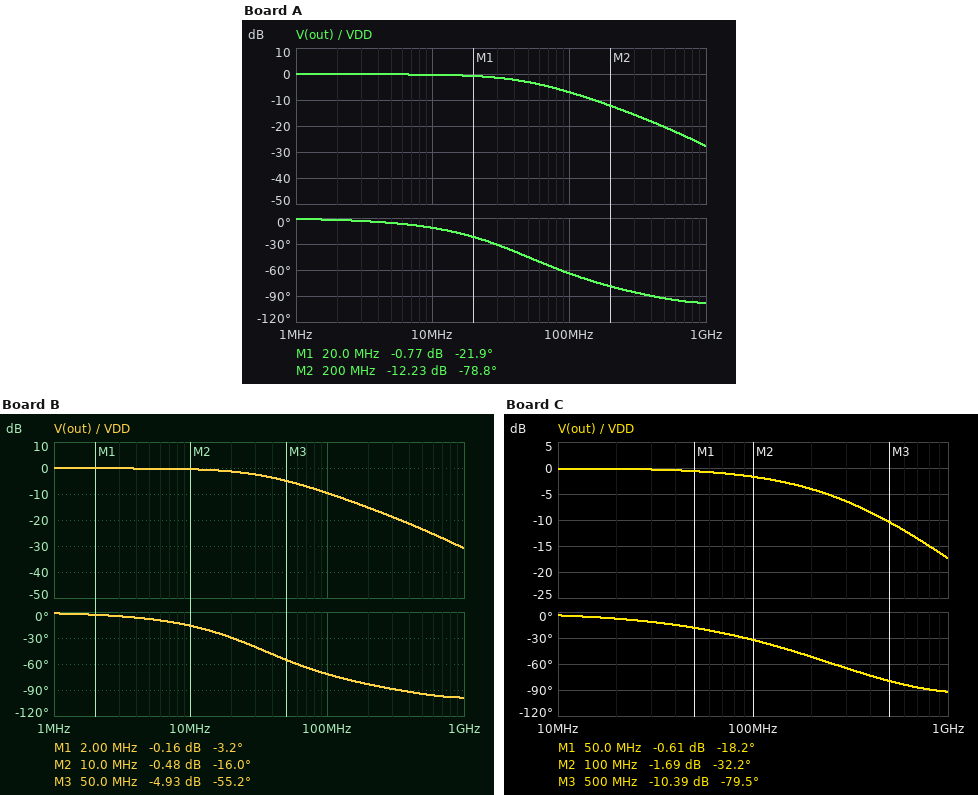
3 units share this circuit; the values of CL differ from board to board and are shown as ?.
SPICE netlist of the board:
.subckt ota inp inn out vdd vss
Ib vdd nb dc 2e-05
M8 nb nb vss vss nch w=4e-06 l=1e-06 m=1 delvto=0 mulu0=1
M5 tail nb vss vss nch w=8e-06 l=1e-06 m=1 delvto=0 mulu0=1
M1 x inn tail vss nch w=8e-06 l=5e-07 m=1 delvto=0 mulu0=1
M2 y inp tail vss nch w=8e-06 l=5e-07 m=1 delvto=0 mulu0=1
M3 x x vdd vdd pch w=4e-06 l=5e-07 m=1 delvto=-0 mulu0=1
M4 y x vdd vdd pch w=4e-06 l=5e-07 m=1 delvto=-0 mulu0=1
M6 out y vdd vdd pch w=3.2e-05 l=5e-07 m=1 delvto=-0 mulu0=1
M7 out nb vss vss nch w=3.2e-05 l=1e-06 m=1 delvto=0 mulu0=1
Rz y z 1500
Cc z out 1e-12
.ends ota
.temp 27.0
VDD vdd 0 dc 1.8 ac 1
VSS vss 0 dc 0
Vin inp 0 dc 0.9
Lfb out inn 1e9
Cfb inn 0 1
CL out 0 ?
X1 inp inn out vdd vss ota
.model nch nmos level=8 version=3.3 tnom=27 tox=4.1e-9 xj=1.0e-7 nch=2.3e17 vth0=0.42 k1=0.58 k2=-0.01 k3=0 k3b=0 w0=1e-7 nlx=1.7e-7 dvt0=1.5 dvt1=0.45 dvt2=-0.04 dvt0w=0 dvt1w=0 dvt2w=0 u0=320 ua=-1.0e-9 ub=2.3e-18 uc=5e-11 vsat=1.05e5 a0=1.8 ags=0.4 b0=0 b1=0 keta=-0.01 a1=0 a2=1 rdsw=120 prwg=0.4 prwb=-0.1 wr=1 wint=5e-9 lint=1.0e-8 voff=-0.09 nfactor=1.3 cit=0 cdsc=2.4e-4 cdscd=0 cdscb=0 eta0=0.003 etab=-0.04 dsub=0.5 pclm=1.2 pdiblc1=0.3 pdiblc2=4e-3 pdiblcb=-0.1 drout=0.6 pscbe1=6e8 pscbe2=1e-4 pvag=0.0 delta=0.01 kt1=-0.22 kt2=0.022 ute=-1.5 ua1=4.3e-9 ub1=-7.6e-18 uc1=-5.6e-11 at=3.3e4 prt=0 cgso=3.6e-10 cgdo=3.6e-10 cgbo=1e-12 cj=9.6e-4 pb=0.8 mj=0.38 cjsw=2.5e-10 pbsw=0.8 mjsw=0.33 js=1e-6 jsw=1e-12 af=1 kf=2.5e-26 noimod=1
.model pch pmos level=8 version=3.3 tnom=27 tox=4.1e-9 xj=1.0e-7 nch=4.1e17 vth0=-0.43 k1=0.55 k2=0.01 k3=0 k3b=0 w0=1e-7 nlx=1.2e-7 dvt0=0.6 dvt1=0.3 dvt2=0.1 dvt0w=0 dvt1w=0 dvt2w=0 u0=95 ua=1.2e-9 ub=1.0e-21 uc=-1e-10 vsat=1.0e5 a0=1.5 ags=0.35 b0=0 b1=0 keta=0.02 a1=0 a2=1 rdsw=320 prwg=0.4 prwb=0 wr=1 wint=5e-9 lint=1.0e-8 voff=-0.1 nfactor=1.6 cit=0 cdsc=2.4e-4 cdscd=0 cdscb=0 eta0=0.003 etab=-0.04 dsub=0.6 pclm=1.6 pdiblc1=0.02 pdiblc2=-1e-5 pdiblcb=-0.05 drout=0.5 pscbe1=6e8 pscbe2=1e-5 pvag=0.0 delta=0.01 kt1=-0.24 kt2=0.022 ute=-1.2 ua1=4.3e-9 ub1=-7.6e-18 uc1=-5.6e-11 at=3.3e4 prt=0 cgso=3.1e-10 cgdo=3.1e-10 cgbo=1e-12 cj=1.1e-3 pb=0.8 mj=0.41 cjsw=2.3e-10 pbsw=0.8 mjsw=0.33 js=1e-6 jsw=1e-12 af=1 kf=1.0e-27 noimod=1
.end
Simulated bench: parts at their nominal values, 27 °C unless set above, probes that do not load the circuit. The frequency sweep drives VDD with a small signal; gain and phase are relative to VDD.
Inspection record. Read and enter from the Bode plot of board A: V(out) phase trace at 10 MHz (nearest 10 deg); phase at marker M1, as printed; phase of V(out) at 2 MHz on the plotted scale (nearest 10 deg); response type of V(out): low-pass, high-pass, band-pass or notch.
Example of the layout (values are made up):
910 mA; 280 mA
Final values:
-10 deg; -21.9 deg; 0 deg; low-pass
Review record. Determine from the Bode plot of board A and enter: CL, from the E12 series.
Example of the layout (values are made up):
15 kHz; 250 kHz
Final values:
2.7 pF
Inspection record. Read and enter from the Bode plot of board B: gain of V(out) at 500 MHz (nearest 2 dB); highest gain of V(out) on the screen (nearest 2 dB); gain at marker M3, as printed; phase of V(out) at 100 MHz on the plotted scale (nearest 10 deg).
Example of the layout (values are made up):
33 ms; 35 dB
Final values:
-24 dB; 0 dB; -4.93 dB; -70 deg
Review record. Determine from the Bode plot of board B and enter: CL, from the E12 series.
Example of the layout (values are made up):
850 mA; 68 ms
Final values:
3.9 pF
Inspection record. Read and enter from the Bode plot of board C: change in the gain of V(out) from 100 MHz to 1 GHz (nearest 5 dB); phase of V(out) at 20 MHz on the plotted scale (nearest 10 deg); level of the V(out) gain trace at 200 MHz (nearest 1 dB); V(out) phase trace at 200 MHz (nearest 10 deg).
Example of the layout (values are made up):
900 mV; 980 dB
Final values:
-15 dB; -10 deg; -4 dB; -50 deg
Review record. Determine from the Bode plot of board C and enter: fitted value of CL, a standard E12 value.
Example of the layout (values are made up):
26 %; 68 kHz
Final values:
820 fF
